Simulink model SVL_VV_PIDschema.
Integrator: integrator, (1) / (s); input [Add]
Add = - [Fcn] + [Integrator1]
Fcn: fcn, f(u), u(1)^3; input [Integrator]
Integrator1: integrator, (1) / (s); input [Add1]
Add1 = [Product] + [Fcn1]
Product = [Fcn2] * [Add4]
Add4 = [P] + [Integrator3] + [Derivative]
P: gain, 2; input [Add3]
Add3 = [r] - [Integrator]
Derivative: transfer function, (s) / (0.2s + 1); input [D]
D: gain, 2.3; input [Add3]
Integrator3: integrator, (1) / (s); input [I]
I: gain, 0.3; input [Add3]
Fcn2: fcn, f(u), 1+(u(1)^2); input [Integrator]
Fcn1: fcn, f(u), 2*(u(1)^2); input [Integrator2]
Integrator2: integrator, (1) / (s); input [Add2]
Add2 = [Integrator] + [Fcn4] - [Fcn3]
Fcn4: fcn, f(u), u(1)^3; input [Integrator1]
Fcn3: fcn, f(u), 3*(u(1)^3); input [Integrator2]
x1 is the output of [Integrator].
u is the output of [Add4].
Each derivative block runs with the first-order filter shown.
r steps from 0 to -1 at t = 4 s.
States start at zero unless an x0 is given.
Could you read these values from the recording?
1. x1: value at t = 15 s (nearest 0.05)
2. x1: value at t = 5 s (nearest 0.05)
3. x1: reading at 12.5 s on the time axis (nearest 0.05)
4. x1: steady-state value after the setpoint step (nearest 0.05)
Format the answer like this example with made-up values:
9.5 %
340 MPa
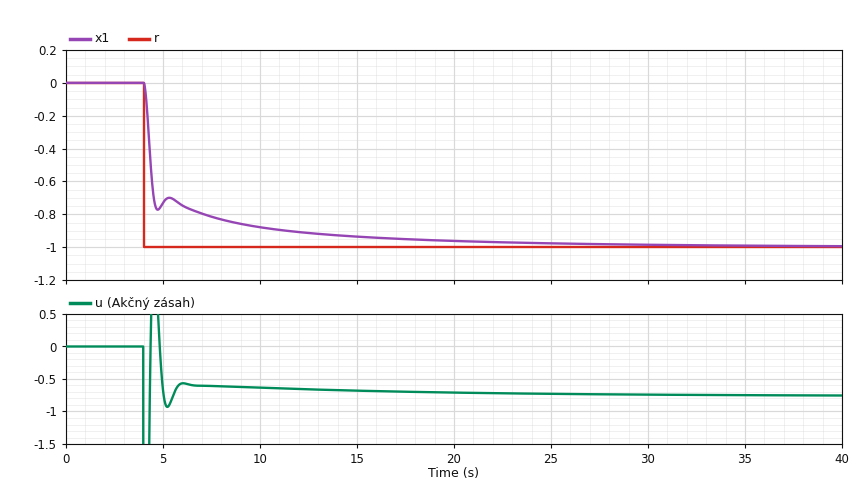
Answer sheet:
-0.95
-0.75
-0.90
-1.00
